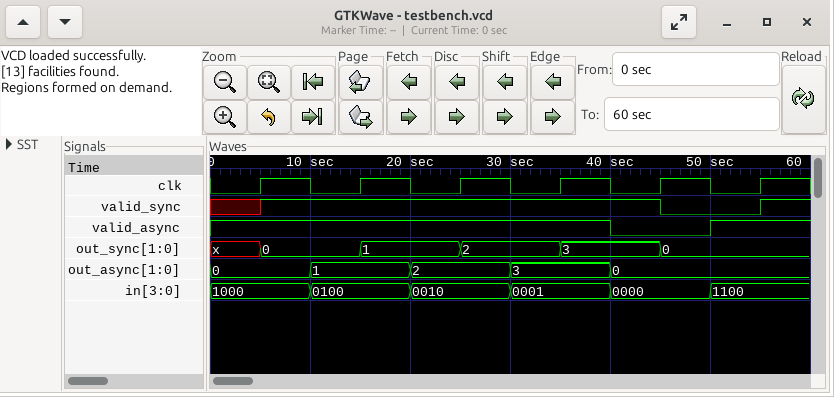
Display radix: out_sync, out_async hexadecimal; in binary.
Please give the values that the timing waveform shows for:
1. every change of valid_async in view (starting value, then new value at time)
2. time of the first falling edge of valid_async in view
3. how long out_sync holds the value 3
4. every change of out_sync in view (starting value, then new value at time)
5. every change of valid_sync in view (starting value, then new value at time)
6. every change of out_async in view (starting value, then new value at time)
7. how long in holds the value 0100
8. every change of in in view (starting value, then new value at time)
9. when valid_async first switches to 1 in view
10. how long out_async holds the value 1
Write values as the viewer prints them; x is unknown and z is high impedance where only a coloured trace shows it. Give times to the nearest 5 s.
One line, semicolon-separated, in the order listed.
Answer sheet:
1, 0 at 40 s, 1 at 50 s; 40 s; 10 s; x, 0 at 5 s, 1 at 15 s, 2 at 25 s, 3 at 35 s, 0 at 45 s; x, 1 at 5 s, 0 at 45 s, 1 at 55 s; 0, 1 at 10 s, 2 at 20 s, 3 at 30 s, 0 at 40 s; 10 s; 1000, 0100 at 10 s, 0010 at 20 s, 0001 at 30 s, 0000 at 40 s, 1100 at 50 s; 50 s; 10 s
